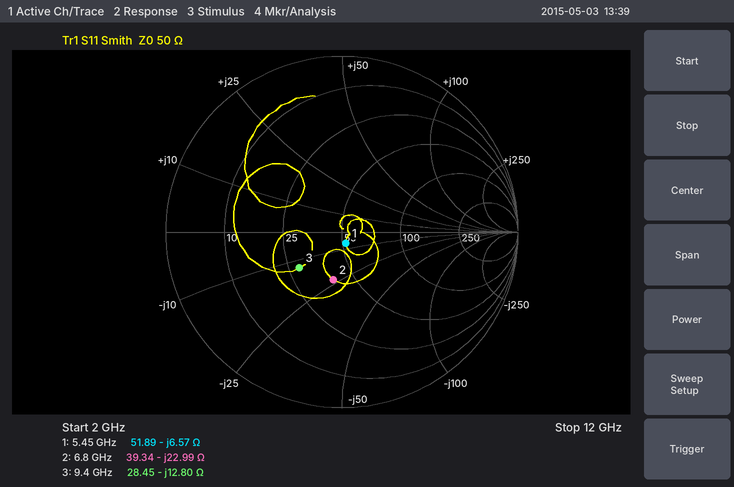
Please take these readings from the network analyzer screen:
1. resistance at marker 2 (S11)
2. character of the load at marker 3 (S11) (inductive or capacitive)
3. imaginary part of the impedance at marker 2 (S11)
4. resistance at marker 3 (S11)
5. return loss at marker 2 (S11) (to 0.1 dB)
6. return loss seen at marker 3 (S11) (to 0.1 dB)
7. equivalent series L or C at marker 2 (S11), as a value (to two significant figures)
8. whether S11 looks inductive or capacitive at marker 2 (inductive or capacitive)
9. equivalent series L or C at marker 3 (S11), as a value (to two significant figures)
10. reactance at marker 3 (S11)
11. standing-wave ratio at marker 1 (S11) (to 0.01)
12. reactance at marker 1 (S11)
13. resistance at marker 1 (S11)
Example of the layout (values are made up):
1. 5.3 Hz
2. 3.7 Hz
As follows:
1. 39.34 Ω
2. capacitive
3. -22.99 Ω
4. 28.45 Ω
5. 11.2 dB
6. 10.0 dB
7. 1.0 pF
8. capacitive
9. 1.3 pF
10. -12.80 Ω
11. 1.14
12. -6.57 Ω
13. 51.89 Ω
